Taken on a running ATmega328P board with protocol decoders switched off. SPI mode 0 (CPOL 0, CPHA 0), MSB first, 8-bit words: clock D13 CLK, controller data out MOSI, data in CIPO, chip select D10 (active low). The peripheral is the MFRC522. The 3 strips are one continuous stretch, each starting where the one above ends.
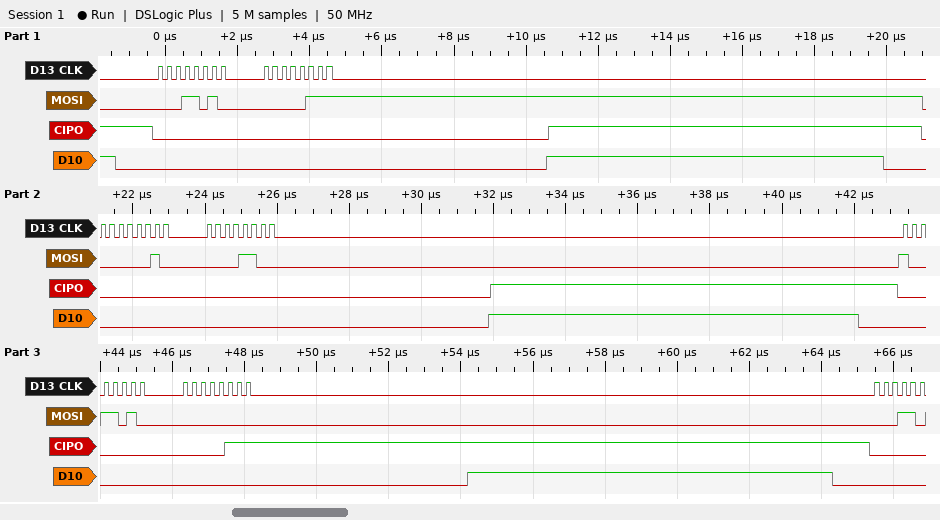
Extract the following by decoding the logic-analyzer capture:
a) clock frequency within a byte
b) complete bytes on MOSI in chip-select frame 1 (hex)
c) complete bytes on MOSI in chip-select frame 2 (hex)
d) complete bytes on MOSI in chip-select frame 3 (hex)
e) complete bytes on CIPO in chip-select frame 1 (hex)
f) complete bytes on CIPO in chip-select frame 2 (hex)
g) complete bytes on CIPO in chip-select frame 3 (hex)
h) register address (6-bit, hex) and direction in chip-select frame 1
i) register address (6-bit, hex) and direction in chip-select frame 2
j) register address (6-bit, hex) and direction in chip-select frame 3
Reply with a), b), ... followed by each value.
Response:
a) 4 MHz
b) 0x1A 0x07
c) 0x02 0x0C
d) 0x9A 0x00
e) 0x00 0x00
f) 0x00 0x00
g) 0x00 0x07
h) 0x0D write
i) 0x01 write
j) 0x0D read
